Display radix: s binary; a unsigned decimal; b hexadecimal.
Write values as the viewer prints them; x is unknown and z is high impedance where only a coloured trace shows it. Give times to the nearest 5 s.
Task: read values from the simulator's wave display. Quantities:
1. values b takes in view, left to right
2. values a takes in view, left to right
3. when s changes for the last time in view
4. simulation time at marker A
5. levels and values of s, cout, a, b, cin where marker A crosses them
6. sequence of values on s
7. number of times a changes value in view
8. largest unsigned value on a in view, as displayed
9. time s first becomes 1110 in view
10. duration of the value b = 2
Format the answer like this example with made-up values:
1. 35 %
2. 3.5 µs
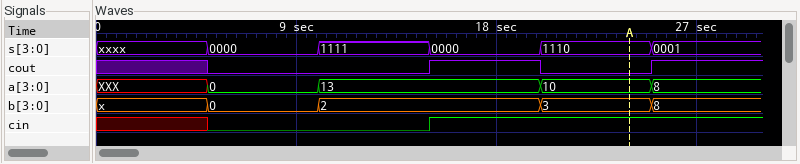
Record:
1. x, 0, 2, 3, 8
2. XXX, 0, 13, 10, 8
3. 25 s
4. 25 s
5. s=1110, cout=0, a=10, b=3, cin=1
6. xxxx, 0000, 1111, 0000, 1110, 0001
7. 4
8. 13
9. 20 s
10. 10 s
